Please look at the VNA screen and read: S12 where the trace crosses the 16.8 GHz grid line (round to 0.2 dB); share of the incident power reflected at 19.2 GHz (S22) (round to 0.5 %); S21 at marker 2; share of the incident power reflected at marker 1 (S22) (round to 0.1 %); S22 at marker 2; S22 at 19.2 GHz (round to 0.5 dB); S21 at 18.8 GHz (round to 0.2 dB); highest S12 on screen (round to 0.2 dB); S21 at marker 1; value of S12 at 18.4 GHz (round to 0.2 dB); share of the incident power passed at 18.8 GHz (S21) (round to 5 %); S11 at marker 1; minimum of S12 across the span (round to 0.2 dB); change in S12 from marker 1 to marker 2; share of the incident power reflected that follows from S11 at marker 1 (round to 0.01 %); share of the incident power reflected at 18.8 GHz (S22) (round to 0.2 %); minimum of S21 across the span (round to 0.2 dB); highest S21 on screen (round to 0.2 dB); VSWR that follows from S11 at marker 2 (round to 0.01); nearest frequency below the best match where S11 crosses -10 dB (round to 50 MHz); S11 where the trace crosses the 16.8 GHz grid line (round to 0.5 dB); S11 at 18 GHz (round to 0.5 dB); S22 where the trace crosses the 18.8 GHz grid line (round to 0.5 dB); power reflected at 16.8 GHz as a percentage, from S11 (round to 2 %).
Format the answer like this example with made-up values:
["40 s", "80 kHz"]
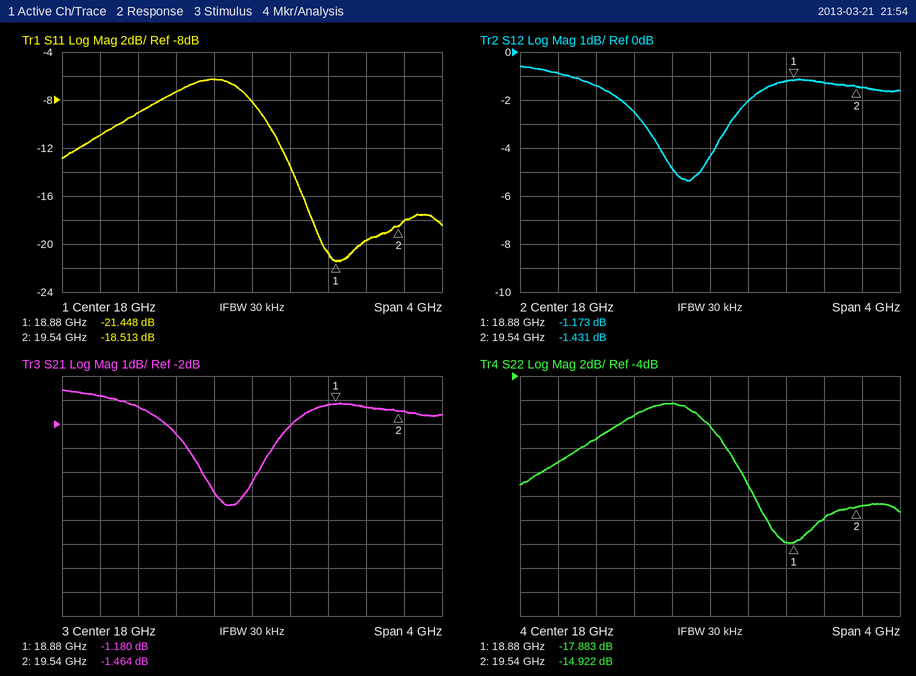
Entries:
["-1.4 dB", "2.5 %", "-1.464 dB", "1.6 %", "-14.922 dB", "-16.0 dB", "-1.2 dB", "-0.6 dB", "-1.180 dB", "-2.0 dB", "75 %", "-21.448 dB", "-5.4 dB", "-0.258 dB", "0.72 %", "1.6 %", "-5.4 dB", "-0.6 dB", "1.27", "18.15 GHz", "-9.0 dB", "-8.0 dB", "-18.0 dB", "12 %"]
